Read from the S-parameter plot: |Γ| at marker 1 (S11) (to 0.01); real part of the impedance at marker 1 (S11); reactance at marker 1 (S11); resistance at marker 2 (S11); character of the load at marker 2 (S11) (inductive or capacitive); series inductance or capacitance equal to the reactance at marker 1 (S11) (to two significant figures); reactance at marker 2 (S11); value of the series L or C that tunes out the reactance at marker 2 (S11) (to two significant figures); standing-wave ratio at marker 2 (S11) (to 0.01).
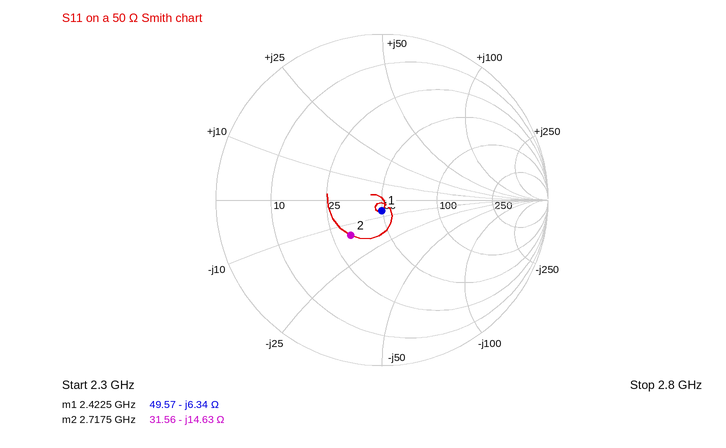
0.06
49.57 Ω
-6.34 Ω
31.56 Ω
capacitive
10 pF
-14.63 Ω
860 pH
1.79
